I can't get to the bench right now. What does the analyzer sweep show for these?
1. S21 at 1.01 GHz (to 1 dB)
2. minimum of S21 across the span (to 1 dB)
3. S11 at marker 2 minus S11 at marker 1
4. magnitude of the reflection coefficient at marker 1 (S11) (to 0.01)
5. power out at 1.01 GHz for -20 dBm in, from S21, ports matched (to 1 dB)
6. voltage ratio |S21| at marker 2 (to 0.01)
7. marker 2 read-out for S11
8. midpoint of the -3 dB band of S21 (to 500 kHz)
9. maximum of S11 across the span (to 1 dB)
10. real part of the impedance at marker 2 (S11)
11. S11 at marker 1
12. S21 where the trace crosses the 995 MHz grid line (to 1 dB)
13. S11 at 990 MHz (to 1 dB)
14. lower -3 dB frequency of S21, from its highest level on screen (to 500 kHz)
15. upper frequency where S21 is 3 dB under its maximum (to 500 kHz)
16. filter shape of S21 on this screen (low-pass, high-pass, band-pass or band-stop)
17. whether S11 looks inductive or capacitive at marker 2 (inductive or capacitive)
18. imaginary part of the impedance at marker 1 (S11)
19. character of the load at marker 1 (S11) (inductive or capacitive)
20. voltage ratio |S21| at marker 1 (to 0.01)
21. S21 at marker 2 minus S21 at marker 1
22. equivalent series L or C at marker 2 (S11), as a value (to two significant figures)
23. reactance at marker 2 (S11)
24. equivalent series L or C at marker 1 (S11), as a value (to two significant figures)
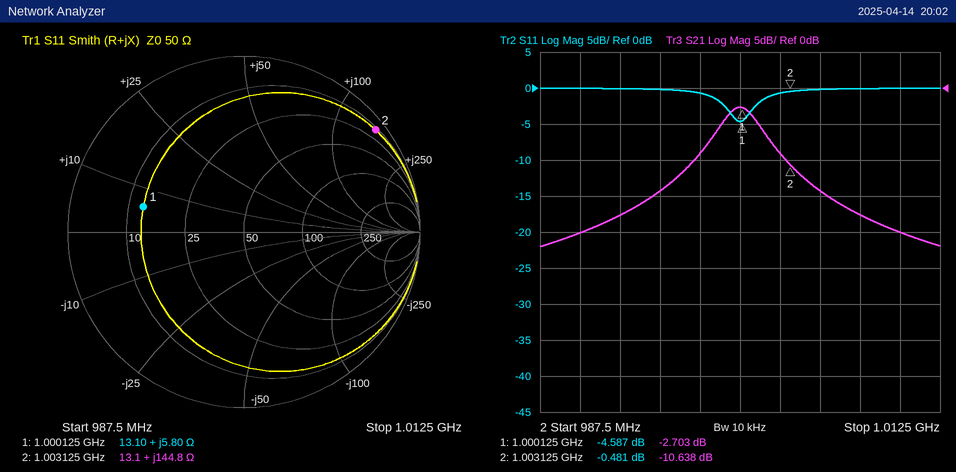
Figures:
-20 dB
-22 dB
4.106 dB
0.59
-40 dBm
0.29
-0.481 dB
1.0000 GHz
0 dB
13.1 Ω
-4.587 dB
-14 dB
0 dB
998.5 MHz
1.0015 GHz
band-pass
inductive
+5.80 Ω
inductive
0.73
-7.935 dB
23 nH
+144.8 Ω
920 pH
